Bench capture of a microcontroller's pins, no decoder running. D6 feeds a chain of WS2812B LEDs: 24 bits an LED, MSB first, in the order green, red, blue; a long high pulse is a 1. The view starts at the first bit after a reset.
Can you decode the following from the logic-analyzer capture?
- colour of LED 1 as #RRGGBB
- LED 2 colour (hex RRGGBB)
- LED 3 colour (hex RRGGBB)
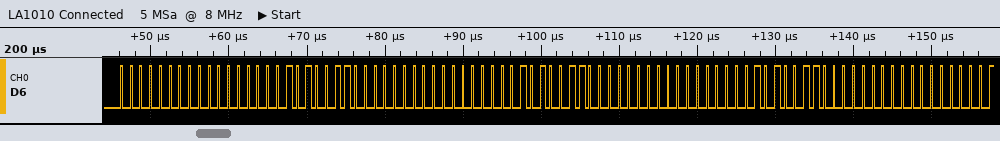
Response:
#000053
#000053
#000053
